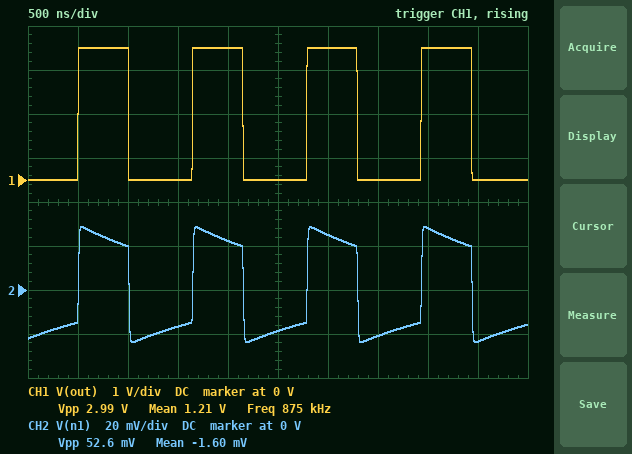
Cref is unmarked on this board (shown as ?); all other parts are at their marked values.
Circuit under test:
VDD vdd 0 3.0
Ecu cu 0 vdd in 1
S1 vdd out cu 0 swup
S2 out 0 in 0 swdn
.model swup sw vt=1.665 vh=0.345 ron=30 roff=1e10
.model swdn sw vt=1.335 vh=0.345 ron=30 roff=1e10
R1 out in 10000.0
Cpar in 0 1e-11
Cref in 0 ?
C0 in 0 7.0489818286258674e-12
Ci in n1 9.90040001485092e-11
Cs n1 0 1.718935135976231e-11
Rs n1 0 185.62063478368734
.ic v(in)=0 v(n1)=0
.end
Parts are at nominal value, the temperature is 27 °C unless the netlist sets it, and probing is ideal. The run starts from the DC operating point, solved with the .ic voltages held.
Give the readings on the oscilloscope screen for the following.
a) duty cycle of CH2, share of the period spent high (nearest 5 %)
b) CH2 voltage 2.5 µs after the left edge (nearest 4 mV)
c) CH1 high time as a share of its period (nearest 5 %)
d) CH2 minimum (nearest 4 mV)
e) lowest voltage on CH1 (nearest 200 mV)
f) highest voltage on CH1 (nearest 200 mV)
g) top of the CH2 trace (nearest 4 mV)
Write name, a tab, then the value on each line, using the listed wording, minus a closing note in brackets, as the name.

duty cycle of CH2, share of the period spent high	45 %
CH2 voltage 2.5 µs after the left edge	-20 mV
CH1 high time as a share of its period	45 %
CH2 minimum	-24 mV
lowest voltage on CH1	0 V
highest voltage on CH1	3.0 V
top of the CH2 trace	28 mV
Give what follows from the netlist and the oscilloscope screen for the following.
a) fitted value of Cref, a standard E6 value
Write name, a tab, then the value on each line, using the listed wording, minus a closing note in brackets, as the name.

fitted value of Cref, a standard E6 value	6.8 pF
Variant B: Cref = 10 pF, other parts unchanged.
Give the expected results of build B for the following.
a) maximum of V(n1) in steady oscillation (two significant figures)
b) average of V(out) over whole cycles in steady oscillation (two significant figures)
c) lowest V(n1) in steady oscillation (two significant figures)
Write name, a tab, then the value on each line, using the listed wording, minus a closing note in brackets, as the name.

maximum of V(n1) in steady oscillation	28 mV
average of V(out) over whole cycles in steady oscillation	1.3 V
lowest V(n1) in steady oscillation	-23 mV
